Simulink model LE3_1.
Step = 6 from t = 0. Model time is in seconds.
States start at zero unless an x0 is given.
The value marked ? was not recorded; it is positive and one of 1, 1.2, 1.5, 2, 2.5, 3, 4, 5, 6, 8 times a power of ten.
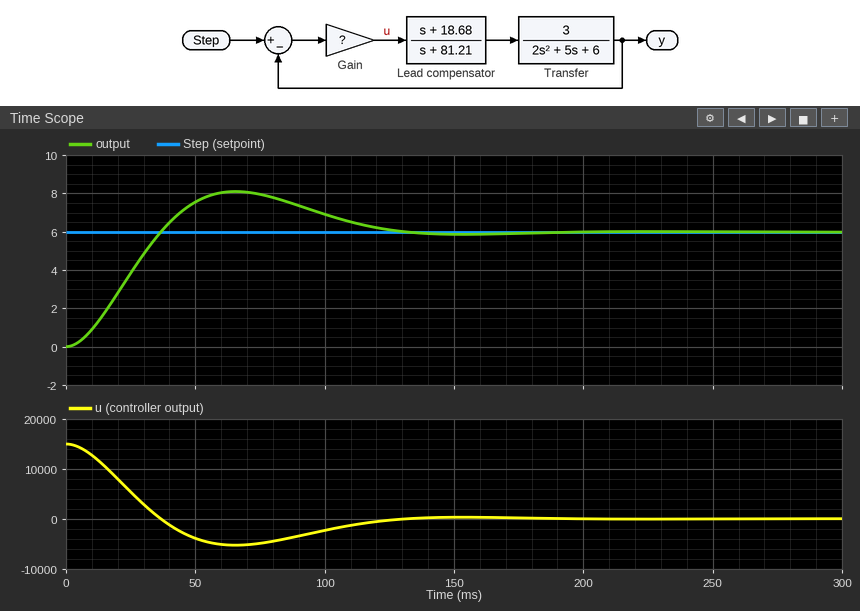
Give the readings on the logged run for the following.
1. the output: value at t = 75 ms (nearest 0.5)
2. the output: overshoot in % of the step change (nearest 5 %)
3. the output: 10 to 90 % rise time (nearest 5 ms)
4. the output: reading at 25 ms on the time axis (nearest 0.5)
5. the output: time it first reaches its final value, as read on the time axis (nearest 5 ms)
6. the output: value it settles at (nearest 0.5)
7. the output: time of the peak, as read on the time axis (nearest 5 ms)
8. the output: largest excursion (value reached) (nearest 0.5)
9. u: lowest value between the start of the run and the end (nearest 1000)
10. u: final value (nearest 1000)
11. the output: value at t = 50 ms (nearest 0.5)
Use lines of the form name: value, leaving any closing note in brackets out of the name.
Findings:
the output: value at t = 75 ms: 8.0
the output: overshoot in % of the step change: 35 %
the output: 10 to 90 % rise time: 25 ms
the output: reading at 25 ms on the time axis: 4.0
the output: time it first reaches its final value, as read on the time axis: 35 ms
the output: value it settles at: 6.0
the output: time of the peak, as read on the time axis: 65 ms
the output: largest excursion (value reached): 8.0
u: lowest value between the start of the run and the end: -5000
u: final value: 0
the output: value at t = 50 ms: 7.5
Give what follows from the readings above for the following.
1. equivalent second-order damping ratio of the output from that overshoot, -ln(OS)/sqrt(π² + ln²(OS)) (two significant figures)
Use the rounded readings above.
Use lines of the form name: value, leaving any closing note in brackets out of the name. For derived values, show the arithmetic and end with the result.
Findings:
equivalent second-order damping ratio of the output from that overshoot, -ln(OS)/sqrt(π² + ln²(OS)): ln(0.35) = -1.050; 1.050 / sqrt(9.870 + 1.102) = 0.32
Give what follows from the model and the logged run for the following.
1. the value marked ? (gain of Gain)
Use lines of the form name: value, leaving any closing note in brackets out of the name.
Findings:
the value marked ?: 2500
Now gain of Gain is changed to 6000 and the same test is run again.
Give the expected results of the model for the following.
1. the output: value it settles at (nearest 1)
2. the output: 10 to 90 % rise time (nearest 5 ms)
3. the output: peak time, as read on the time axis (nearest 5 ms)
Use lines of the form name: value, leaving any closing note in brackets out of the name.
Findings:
the output: value it settles at: 6
the output: 10 to 90 % rise time: 15 ms
the output: peak time, as read on the time axis: 35 ms
